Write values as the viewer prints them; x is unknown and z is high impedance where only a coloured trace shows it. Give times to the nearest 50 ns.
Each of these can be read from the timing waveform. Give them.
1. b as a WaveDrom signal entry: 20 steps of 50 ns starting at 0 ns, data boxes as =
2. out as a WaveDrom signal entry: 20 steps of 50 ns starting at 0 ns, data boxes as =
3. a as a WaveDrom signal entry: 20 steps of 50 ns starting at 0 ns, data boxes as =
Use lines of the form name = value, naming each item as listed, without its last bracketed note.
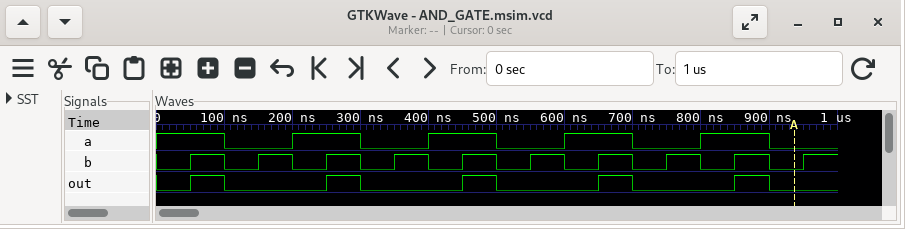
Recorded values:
b as a WaveDrom signal entry: 20 steps of 50 ns starting at 0 ns, data boxes as = = {name: 'b', wave: '01010101010101010101'}
out as a WaveDrom signal entry: 20 steps of 50 ns starting at 0 ns, data boxes as = = {name: 'out', wave: '010..10..10..10..10.'}
a as a WaveDrom signal entry: 20 steps of 50 ns starting at 0 ns, data boxes as = = {name: 'a', wave: '1.0.1.0.1.0.1.0.1.0.'}
